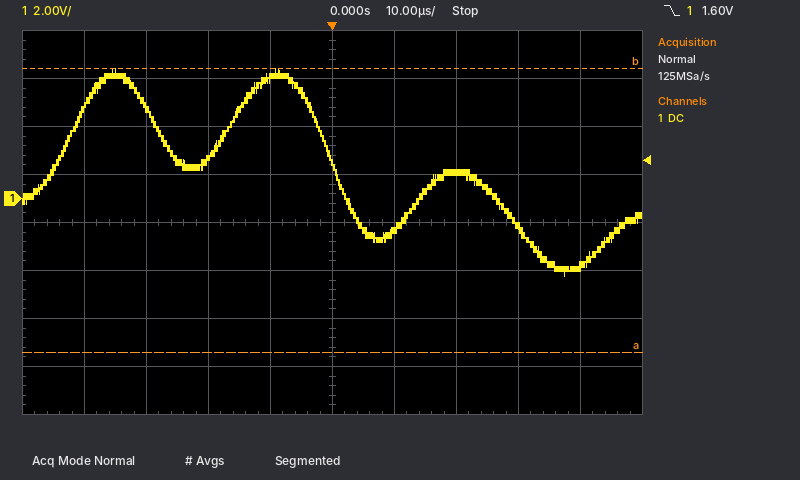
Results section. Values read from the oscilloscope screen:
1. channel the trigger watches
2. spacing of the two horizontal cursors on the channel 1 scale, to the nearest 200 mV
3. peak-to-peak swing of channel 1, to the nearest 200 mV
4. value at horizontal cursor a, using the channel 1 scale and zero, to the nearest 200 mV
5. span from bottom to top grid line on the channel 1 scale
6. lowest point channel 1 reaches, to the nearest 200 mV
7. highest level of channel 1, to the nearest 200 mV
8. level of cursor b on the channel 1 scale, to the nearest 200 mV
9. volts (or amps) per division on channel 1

channel 1
11.8 V
8.6 V
-6.4 V
16 V
-3.2 V
5.4 V
5.4 V
2 V
